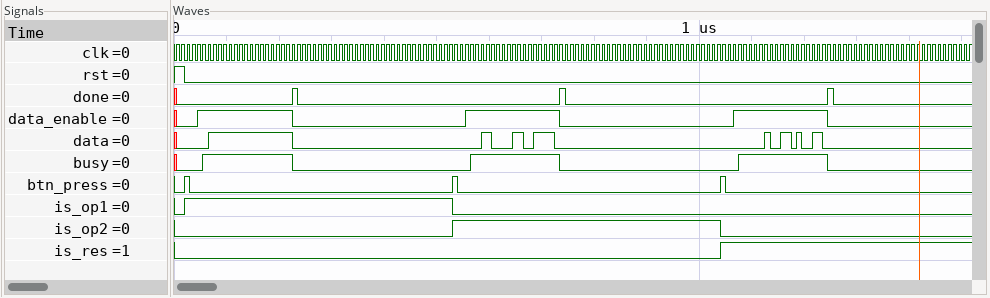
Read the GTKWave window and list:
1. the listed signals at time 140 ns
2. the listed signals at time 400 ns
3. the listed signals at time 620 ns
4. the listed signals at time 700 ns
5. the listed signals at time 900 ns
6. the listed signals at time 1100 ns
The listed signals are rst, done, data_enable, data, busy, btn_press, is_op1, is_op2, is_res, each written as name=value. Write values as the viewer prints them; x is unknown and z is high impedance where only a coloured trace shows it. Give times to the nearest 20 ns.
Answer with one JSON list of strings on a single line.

["rst=0, done=0, data_enable=1, data=1, busy=1, btn_press=0, is_op1=1, is_op2=0, is_res=0", "rst=0, done=0, data_enable=0, data=0, busy=0, btn_press=0, is_op1=1, is_op2=0, is_res=0", "rst=0, done=0, data_enable=1, data=0, busy=1, btn_press=0, is_op1=0, is_op2=1, is_res=0", "rst=0, done=0, data_enable=1, data=1, busy=1, btn_press=0, is_op1=0, is_op2=1, is_res=0", "rst=0, done=0, data_enable=0, data=0, busy=0, btn_press=0, is_op1=0, is_op2=1, is_res=0", "rst=0, done=0, data_enable=1, data=0, busy=1, btn_press=0, is_op1=0, is_op2=0, is_res=1"]
